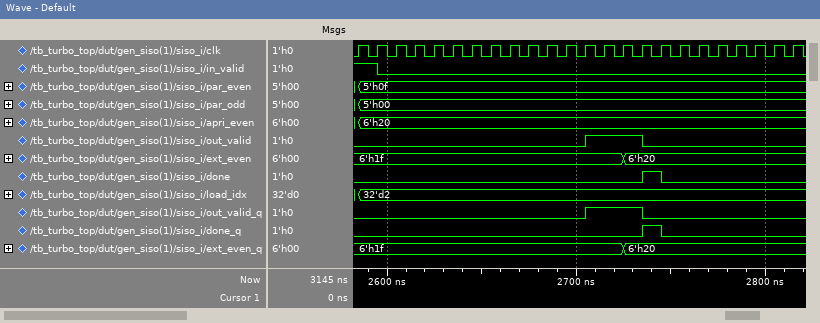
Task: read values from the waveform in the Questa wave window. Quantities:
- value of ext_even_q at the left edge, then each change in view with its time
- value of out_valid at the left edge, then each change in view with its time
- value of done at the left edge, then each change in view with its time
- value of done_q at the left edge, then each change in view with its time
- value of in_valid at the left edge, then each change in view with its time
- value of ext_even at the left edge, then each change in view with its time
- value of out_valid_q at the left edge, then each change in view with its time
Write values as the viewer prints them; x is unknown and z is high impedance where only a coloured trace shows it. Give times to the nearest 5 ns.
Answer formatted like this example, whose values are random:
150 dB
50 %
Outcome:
6'h1f, 6'h20 at 2725 ns
0, 1 at 2705 ns, 0 at 2735 ns
0, 1 at 2735 ns, 0 at 2745 ns
0, 1 at 2735 ns, 0 at 2745 ns
1, 0 at 2595 ns
6'h1f, 6'h20 at 2725 ns
0, 1 at 2705 ns, 0 at 2735 ns
